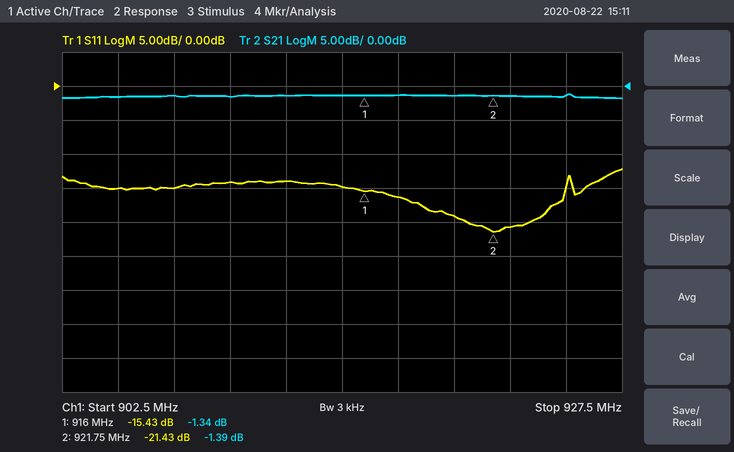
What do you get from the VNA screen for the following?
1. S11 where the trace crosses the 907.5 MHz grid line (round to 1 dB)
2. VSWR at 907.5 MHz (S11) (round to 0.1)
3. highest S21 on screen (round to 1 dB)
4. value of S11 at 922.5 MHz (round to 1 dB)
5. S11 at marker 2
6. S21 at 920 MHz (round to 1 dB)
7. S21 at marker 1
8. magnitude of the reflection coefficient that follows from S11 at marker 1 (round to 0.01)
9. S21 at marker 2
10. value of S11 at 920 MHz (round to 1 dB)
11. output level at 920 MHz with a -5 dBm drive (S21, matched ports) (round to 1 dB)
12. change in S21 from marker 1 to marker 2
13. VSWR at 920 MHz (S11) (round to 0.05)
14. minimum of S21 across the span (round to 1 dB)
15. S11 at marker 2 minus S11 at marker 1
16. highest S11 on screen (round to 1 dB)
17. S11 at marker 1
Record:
-15 dB
1.4
-1 dB
-21 dB
-21.43 dB
-1 dB
-1.34 dB
0.17
-1.39 dB
-19 dB
-6 dBm
-0.05 dB
1.25
-2 dB
-6.00 dB
-12 dB
-15.43 dB
